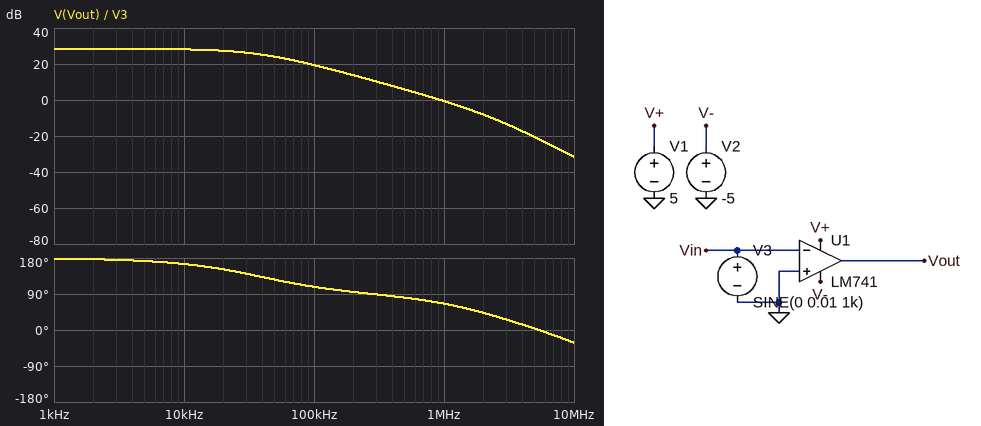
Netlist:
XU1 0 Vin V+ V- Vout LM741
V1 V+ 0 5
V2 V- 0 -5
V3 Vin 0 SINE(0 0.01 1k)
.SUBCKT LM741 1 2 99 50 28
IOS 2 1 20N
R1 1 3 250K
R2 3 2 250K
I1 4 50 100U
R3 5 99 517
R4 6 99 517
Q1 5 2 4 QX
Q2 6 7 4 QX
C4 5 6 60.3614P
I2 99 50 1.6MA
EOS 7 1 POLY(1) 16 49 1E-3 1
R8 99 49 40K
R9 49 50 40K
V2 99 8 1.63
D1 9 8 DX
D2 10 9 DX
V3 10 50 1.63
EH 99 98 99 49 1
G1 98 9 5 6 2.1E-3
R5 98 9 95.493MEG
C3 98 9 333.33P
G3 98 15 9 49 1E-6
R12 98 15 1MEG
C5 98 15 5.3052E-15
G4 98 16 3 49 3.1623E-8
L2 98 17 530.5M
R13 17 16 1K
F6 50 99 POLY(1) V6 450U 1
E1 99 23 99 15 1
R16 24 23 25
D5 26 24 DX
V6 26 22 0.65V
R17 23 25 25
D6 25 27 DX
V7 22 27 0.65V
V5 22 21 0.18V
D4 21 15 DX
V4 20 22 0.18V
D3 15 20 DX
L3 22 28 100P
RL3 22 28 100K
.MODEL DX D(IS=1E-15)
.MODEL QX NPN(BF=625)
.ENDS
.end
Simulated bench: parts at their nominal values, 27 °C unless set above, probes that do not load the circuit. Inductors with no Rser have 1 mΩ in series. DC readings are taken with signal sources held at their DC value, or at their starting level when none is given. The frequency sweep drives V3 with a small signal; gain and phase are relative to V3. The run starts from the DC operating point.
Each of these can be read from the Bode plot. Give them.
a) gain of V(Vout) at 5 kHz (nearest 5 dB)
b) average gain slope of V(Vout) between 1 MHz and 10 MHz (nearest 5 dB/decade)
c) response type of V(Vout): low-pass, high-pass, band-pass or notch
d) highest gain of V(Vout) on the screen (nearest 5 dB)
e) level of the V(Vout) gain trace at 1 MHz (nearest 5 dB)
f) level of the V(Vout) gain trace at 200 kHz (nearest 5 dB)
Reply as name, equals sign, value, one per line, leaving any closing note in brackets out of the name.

gain of V(Vout) at 5 kHz = 30 dB
average gain slope of V(Vout) between 1 MHz and 10 MHz = -30 dB/decade
response type of V(Vout): low-pass, high-pass, band-pass or notch = low-pass
highest gain of V(Vout) on the screen = 30 dB
level of the V(Vout) gain trace at 1 MHz = 0 dB
level of the V(Vout) gain trace at 200 kHz = 15 dB
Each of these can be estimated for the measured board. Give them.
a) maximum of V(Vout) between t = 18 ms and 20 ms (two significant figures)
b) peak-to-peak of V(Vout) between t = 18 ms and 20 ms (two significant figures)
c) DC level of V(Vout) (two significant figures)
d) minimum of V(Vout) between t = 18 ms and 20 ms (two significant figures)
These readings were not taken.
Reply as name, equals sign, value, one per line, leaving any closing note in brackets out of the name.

maximum of V(Vout) between t = 18 ms and 20 ms = 4.0 V
peak-to-peak of V(Vout) between t = 18 ms and 20 ms = 8.0 V
DC level of V(Vout) = 3.9 V
minimum of V(Vout) between t = 18 ms and 20 ms = -4.0 V
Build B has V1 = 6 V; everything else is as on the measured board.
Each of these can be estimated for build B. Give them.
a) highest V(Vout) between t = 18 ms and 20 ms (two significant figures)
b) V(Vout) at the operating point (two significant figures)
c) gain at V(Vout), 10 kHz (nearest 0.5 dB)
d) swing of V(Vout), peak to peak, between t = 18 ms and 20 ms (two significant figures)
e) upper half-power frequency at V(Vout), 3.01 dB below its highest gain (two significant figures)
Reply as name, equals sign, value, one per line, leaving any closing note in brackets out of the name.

highest V(Vout) between t = 18 ms and 20 ms = 5.0 V
V(Vout) at the operating point = 4.9 V
gain at V(Vout), 10 kHz = 28.5 dB
swing of V(Vout), peak to peak, between t = 18 ms and 20 ms = 9.0 V
upper half-power frequency at V(Vout), 3.01 dB below its highest gain = 37 kHz
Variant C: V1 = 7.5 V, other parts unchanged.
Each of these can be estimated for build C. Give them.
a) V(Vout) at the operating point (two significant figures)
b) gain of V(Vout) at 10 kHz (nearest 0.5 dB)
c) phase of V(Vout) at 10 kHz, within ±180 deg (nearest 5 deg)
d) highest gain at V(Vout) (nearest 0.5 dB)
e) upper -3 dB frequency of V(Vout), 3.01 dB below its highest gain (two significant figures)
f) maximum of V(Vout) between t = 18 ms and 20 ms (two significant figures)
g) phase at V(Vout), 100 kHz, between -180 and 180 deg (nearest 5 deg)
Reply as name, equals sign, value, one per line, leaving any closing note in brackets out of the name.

V(Vout) at the operating point = 6.4 V
gain of V(Vout) at 10 kHz = 28.5 dB
phase of V(Vout) at 10 kHz, within ±180 deg = 165 deg
highest gain at V(Vout) = 29.0 dB
upper -3 dB frequency of V(Vout), 3.01 dB below its highest gain = 36 kHz
maximum of V(Vout) between t = 18 ms and 20 ms = 6.5 V
phase at V(Vout), 100 kHz, between -180 and 180 deg = 105 deg
